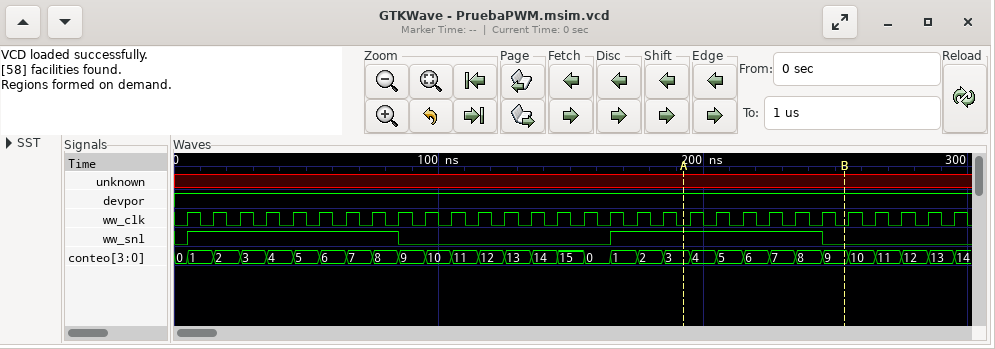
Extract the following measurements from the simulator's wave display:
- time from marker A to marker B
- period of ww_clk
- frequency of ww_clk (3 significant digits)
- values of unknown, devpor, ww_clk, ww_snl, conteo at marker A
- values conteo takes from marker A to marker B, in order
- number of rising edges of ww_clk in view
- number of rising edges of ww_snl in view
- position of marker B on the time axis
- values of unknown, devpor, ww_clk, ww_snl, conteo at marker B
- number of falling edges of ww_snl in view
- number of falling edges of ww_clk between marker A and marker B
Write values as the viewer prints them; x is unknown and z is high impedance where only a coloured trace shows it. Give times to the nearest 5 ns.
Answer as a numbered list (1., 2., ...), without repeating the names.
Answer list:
1. 60 ns
2. 10 ns
3. 100 MHz
4. unknown=x, devpor=1, ww_clk=0, ww_snl=1, conteo=3
5. 3, 4, 5, 6, 7, 8, 9
6. 30
7. 2
8. 255 ns
9. unknown=x, devpor=1, ww_clk=0, ww_snl=0, conteo=9
10. 2
11. 6
